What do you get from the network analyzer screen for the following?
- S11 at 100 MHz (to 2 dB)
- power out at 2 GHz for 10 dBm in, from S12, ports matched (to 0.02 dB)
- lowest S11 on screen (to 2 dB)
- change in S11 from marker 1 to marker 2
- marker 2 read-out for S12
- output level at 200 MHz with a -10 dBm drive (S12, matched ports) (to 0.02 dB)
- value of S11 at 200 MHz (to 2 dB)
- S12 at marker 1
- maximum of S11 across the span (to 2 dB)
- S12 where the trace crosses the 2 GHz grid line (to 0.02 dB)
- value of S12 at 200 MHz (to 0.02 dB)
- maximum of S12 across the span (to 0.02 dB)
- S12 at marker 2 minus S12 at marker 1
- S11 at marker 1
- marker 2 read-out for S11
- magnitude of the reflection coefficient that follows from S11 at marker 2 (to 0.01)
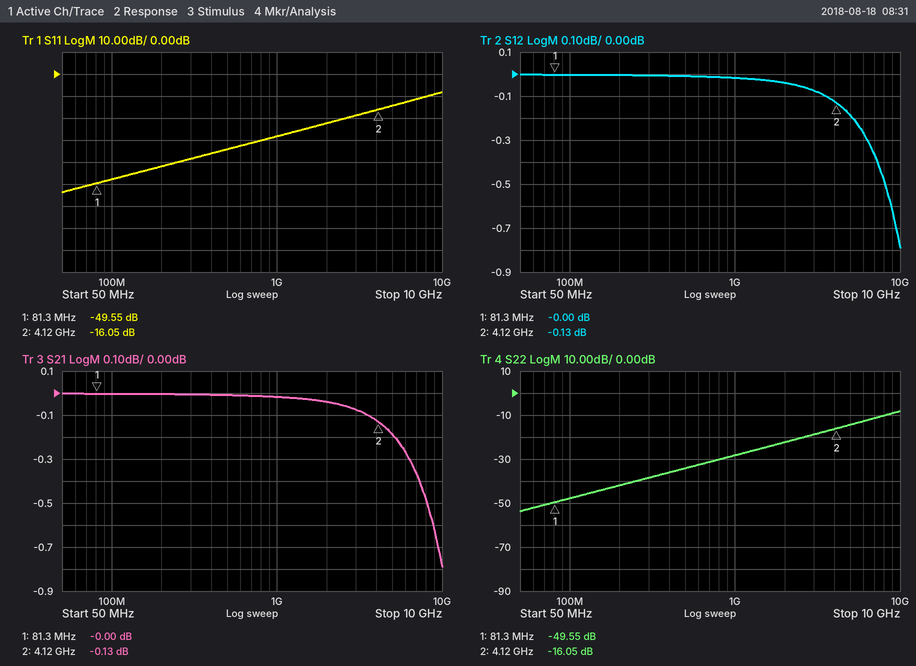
-48 dB
9.96 dBm
-54 dB
33.50 dB
-0.13 dB
-10.00 dBm
-42 dB
-0.00 dB
-8 dB
-0.04 dB
0.00 dB
0.00 dB
-0.13 dB
-49.55 dB
-16.05 dB
0.16
